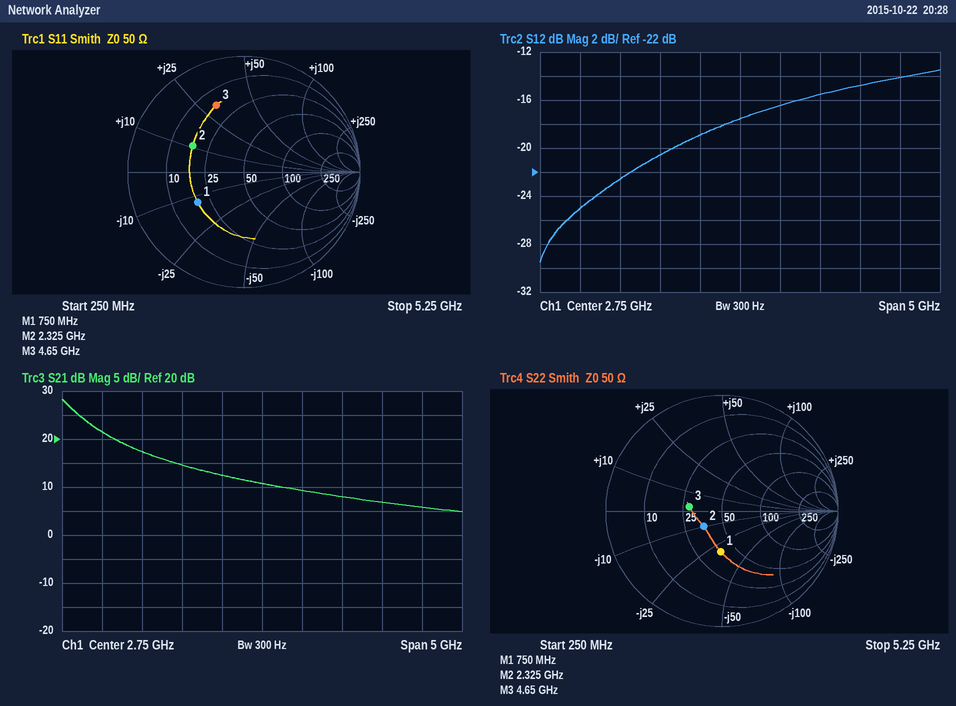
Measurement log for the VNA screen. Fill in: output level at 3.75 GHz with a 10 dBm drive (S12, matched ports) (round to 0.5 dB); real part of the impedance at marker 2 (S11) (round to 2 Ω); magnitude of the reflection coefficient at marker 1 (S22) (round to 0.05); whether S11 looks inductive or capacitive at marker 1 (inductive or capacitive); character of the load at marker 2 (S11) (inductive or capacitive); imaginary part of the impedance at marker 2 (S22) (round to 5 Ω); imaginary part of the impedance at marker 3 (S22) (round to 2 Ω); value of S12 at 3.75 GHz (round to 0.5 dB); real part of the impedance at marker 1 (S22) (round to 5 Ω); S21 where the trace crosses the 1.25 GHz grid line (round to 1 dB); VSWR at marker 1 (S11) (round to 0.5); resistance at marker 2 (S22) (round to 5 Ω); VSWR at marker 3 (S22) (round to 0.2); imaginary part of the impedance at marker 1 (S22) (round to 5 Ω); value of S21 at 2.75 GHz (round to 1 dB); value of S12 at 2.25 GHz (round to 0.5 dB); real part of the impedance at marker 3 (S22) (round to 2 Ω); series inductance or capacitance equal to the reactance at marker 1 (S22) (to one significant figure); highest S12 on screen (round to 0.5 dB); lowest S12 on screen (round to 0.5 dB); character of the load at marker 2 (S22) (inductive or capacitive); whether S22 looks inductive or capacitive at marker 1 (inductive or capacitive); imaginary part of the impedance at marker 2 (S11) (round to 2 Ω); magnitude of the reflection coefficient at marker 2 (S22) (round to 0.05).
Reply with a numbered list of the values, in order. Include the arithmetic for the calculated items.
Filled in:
1. 10 dBm + (-15.5 dB) = -5.5 dBm
2. 18 Ω
3. 0.35
4. capacitive
5. inductive
6. -10 Ω
7. +2 Ω
8. -15.5 dB
9. 40 Ω
10. 17 dB
11. 3.0
12. 35 Ω
13. 1.8
14. -30 Ω
15. 11 dB
16. -19.0 dB
17. 28 Ω
18. C = 1/(2π × 750 MHz × 30 Ω) ≈ 7 pF
19. -13.5 dB
20. -29.5 dB
21. capacitive
22. capacitive
23. +10 Ω
24. 0.20
